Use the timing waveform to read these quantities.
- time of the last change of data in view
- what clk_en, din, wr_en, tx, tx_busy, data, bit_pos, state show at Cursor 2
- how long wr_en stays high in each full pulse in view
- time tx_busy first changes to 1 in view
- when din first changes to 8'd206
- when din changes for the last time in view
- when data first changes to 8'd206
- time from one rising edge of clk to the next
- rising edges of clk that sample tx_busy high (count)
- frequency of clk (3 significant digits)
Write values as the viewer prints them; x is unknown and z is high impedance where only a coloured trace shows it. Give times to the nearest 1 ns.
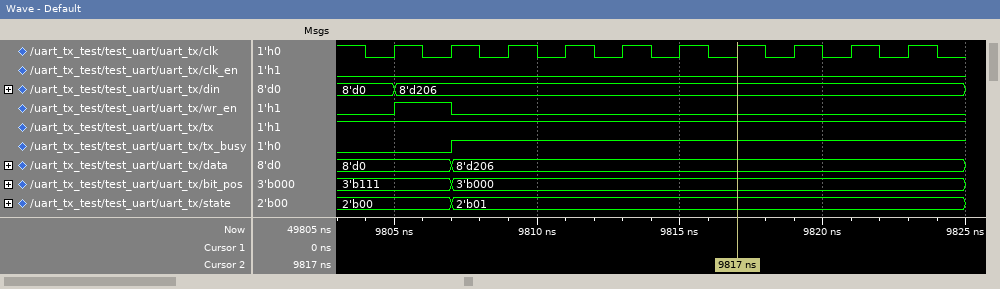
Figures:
9807 ns
clk_en=0, din=8'd206, wr_en=0, tx=1, tx_busy=1, data=8'd206, bit_pos=3'b000, state=2'b01
2 ns
9807 ns
9805 ns
9805 ns
9807 ns
2 ns
8
500 MHz
